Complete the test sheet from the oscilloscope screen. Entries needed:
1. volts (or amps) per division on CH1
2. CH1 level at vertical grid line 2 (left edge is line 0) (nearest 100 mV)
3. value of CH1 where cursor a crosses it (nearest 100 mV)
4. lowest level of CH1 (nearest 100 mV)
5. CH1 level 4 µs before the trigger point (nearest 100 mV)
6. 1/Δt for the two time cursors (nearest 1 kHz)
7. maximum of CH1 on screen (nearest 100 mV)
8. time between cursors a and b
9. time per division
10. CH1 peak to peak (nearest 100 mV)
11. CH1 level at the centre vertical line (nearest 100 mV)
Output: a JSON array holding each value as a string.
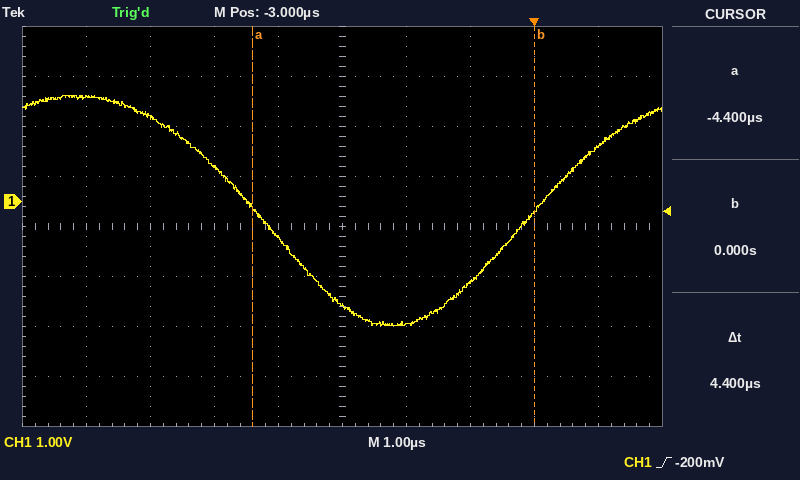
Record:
["1 V", "1.7 V", "-100 mV", "-2.5 V", "-700 mV", "227 kHz", "2.1 V", "4.4 µs", "1 µs", "4.6 V", "-2.1 V"]
